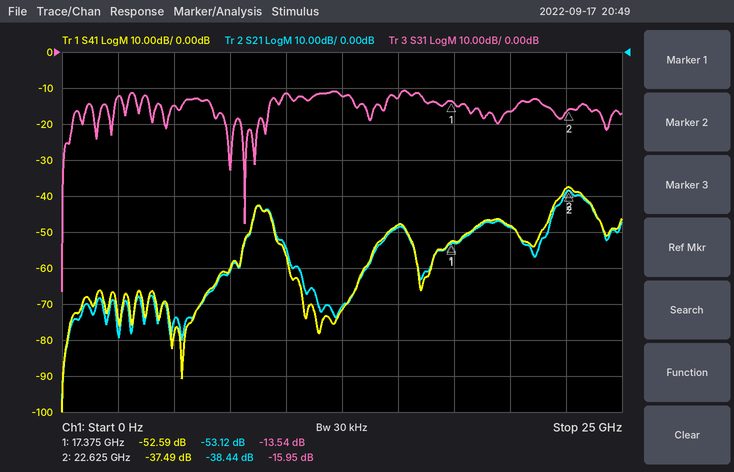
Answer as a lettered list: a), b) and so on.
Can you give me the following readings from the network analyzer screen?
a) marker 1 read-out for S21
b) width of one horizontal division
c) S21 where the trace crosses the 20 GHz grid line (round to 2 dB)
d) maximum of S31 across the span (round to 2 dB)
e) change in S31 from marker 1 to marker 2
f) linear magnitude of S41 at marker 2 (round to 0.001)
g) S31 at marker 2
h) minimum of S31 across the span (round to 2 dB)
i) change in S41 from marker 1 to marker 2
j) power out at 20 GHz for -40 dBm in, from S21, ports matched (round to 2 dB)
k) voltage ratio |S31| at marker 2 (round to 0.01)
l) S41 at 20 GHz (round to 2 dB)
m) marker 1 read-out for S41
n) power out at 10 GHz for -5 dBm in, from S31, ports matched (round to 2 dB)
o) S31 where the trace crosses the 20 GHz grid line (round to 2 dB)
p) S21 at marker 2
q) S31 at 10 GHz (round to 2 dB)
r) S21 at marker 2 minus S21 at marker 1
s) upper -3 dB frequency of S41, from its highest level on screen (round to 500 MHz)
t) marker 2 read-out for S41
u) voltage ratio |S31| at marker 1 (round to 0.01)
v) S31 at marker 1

a) -53.12 dB
b) 2.5 GHz
c) -48 dB
d) -10 dB
e) -2.41 dB
f) 0.013
g) -15.95 dB
h) -66 dB
i) 15.10 dB
j) -88 dBm
k) 0.16
l) -48 dB
m) -52.59 dB
n) -16 dBm
o) -16 dB
p) -38.44 dB
q) -12 dB
r) 14.68 dB
s) 23.5 GHz
t) -37.49 dB
u) 0.21
v) -13.54 dB
